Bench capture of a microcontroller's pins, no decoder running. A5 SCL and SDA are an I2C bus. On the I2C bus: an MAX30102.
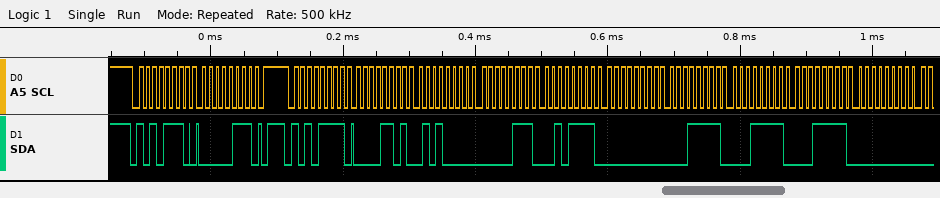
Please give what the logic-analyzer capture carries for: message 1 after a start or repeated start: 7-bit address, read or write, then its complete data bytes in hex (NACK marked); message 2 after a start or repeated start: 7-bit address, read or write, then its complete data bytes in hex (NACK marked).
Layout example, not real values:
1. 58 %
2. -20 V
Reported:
1. 0x57 write: 07
2. 0x57 read: 0D 50 07 2F 00 1F 1F 1F 00
